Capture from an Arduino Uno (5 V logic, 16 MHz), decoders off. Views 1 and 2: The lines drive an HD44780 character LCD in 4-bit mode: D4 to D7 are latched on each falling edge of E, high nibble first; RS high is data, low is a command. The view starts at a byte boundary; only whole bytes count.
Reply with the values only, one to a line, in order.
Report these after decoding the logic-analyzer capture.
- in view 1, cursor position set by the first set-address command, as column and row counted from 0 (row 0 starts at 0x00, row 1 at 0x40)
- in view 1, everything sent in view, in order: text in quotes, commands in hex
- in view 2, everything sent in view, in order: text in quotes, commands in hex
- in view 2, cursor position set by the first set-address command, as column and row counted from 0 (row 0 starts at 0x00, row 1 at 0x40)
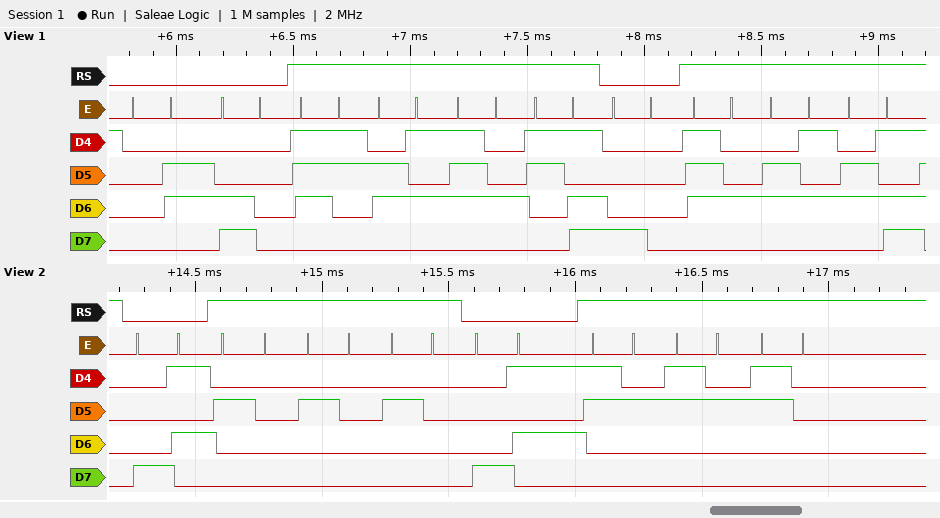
column 0, row 1
0x06 0xC0 "set=" 0x80 "tem"
0x85 "   " 0x85 "220"
column 5, row 0
